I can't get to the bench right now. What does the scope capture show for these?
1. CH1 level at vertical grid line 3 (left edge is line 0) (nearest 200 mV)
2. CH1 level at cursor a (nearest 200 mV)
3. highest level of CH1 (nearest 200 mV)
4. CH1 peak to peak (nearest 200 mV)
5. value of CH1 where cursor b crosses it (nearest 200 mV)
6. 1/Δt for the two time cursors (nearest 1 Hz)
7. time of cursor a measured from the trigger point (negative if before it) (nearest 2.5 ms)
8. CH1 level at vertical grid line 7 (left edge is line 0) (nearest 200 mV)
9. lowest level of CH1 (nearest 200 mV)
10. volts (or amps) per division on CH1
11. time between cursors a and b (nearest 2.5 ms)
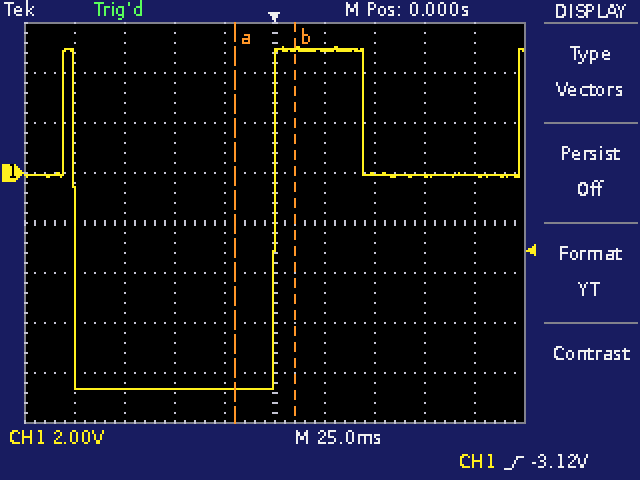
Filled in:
-8.6 V
-8.6 V
5.0 V
13.6 V
5.0 V
33 Hz
-20.0 ms
0.0 V
-8.6 V
2 V
30.0 ms
